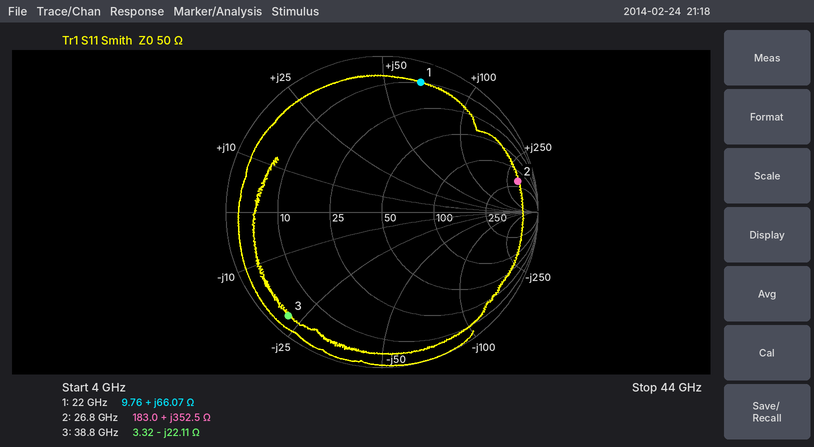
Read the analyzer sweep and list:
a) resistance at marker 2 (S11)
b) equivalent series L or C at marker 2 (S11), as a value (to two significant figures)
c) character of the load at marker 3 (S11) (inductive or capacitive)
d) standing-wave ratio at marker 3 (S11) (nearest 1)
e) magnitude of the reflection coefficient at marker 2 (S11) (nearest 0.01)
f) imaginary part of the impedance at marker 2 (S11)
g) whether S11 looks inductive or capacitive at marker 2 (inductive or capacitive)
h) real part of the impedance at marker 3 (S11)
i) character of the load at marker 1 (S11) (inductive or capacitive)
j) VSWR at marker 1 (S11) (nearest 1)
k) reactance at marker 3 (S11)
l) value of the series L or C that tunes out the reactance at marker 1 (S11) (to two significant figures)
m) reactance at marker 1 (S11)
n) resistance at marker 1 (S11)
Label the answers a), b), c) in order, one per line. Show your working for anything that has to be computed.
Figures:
a) 183.0 Ω
b) L = 352.5 Ω/(2π × 26.8 GHz) ≈ 2.1 nH
c) capacitive
d) 18
e) 0.89
f) +352.5 Ω
g) inductive
h) 3.32 Ω
i) inductive
j) 14
k) -22.11 Ω
l) C = 1/(2π × 22 GHz × 66.07 Ω) ≈ 109 fF, so 110 fF to two significant figures
m) +66.07 Ω
n) 9.76 Ω
